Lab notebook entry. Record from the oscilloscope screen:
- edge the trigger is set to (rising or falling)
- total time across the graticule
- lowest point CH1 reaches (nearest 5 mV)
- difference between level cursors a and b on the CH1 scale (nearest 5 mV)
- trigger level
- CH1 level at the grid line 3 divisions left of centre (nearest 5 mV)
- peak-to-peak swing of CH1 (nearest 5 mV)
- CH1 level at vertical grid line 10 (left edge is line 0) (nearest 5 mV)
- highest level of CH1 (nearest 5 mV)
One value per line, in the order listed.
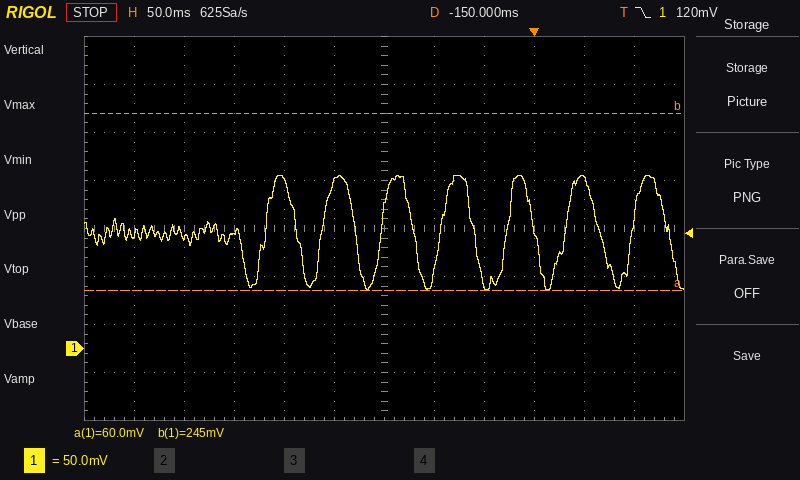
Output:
falling
600 ms
60 mV
185 mV
120 mV
120 mV
120 mV
175 mV
180 mV
